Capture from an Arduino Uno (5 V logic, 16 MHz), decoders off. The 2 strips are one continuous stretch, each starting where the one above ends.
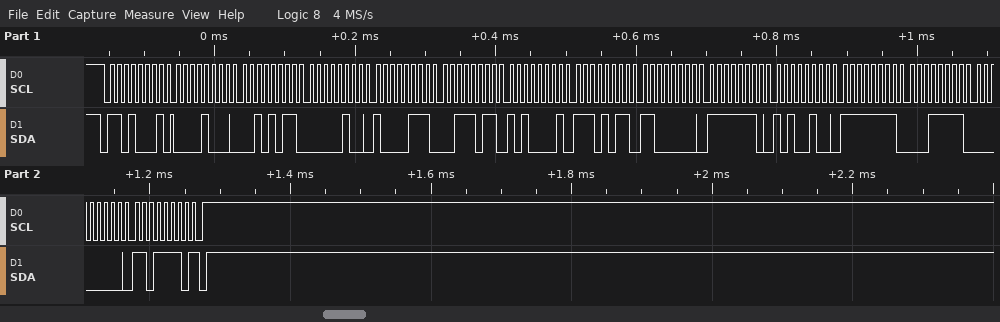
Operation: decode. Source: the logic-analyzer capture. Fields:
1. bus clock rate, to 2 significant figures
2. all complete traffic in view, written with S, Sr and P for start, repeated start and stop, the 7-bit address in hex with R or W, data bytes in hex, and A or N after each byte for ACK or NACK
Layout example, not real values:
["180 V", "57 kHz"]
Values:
["100 kHz", "S 68R A 08 A 2B A 04 A 87 A 3B A A1 A EB A C0 A FE A A4 A FF A 1F A 00 A DE N P"]
